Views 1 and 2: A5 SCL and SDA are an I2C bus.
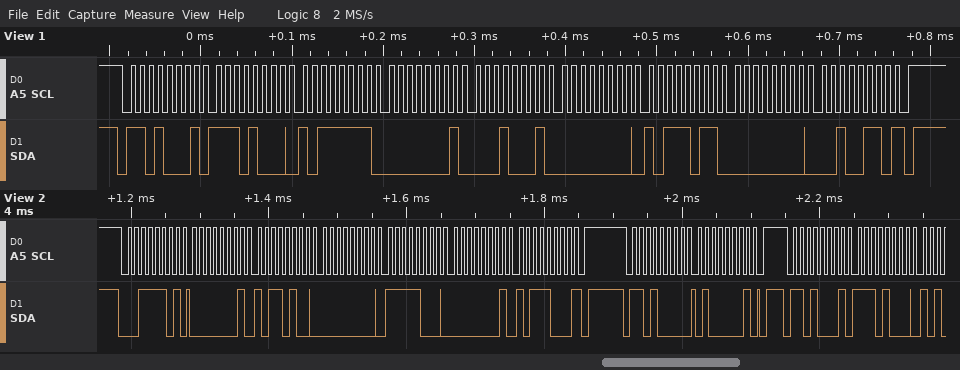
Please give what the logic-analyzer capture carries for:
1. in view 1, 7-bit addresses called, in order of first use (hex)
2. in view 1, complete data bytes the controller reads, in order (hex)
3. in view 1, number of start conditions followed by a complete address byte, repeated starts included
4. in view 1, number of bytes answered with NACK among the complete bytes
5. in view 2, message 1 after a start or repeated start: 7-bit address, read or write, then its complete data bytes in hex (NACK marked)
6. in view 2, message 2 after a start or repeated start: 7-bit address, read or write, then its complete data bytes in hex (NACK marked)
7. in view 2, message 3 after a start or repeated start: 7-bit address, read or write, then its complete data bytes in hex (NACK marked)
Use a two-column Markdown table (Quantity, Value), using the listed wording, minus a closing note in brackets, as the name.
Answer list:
| Quantity | Value |
|---|---|
| in view 1, 7-bit addresses called, in order of first use | 0x68 |
| in view 1, complete data bytes the controller reads, in order | E8 BF 01 11 00 BB 00 26 |
| in view 1, number of start conditions followed by a complete address byte, repeated starts included | 1 |
| in view 1, number of bytes answered with NACK among the complete bytes | 1 |
| in view 2, message 1 after a start or repeated start: 7-bit address, read or write, then its complete data bytes in hex | 0x1E read: 01 B4 00 F8 01 B8 NACK |
| in view 2, message 2 after a start or repeated start: 7-bit address, read or write, then its complete data bytes in hex | 0x68 write: 41 |
| in view 2, message 3 after a start or repeated start: 7-bit address, read or write, then its complete data bytes in hex | 0x68 read: E8 |
